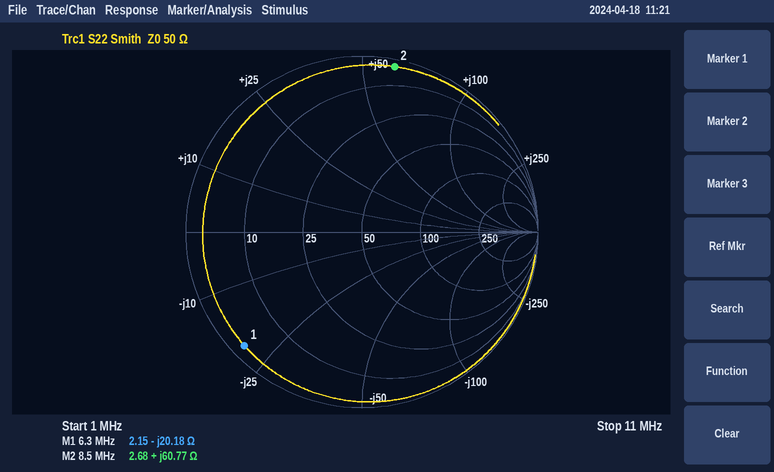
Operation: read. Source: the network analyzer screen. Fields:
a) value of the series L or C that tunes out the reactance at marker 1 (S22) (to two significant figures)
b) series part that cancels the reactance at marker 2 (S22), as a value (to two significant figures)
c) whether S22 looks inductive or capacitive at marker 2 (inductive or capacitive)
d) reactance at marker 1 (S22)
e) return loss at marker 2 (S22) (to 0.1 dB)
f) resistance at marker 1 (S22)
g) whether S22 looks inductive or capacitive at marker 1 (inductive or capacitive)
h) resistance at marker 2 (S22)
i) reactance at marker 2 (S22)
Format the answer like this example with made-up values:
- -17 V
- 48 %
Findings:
- 510 nH
- 310 pF
- inductive
- -20.18 Ω
- 0.4 dB
- 2.15 Ω
- capacitive
- 2.68 Ω
- +60.77 Ω
